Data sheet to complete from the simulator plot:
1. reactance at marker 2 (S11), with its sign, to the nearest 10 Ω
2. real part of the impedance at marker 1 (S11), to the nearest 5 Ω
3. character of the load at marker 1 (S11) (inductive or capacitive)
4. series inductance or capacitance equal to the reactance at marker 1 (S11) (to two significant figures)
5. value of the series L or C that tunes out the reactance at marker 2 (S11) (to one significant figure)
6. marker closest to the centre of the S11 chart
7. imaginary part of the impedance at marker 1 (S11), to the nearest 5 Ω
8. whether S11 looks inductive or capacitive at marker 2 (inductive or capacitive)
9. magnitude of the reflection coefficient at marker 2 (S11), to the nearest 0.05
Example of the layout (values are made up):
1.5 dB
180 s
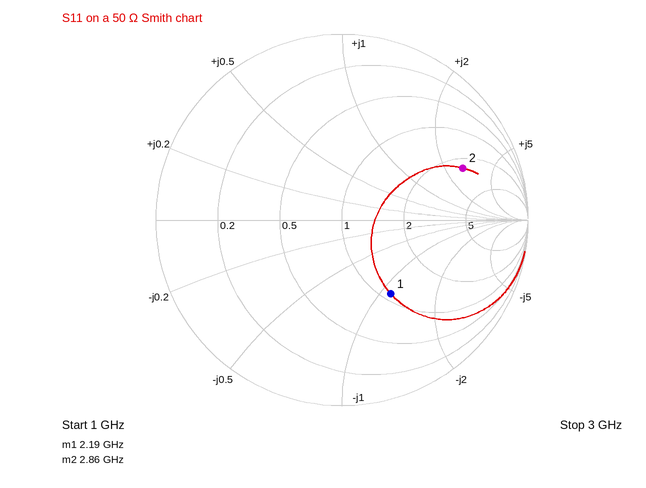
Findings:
+140 Ω
55 Ω
capacitive
1.3 pF
400 fF
marker 1
-55 Ω
inductive
0.70
